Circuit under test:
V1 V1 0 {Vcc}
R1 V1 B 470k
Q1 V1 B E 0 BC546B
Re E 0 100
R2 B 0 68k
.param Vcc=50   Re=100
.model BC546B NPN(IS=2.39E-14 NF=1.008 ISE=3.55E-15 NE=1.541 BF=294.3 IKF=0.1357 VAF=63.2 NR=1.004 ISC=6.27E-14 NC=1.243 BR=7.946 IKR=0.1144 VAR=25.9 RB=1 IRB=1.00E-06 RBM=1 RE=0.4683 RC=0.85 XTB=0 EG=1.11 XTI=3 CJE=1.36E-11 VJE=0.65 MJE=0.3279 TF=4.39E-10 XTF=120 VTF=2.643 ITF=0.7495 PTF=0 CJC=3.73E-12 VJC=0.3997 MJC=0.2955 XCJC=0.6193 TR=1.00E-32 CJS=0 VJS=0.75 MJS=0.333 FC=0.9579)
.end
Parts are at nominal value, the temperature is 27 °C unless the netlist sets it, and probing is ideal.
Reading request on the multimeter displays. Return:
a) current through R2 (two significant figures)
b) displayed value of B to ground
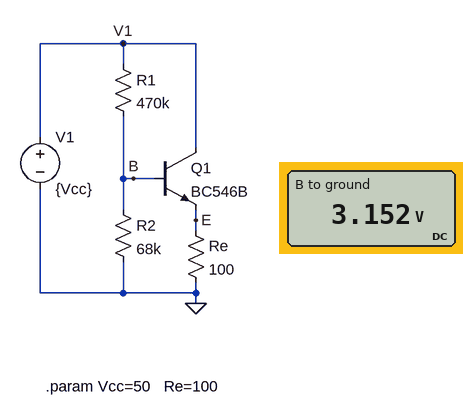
46 µA
3.152 V
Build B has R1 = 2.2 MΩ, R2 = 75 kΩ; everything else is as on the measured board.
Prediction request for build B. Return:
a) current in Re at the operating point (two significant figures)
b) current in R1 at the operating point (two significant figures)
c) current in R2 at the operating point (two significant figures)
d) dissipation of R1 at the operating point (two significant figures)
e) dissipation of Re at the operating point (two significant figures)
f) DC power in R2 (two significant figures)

4.0 mA
22 µA
14 µA
1.1 mW
1.6 mW
15 µW
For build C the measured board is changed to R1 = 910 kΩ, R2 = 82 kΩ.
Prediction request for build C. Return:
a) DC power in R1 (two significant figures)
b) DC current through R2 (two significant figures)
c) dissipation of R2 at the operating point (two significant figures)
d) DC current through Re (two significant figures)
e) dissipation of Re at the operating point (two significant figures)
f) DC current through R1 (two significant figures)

2.5 mW
25 µA
51 µW
13 mA
18 mW
53 µA
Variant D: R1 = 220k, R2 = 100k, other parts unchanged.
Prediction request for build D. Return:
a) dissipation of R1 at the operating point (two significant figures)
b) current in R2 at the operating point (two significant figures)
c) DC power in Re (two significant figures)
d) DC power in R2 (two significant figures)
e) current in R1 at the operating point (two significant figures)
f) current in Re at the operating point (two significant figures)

8.7 mW
62 µA
290 mW
380 µW
200 µA
54 mA
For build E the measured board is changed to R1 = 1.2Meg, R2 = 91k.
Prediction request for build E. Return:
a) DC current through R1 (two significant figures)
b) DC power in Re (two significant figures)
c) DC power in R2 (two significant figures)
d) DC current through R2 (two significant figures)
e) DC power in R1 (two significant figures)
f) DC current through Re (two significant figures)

40 µA
11 mW
33 µW
19 µA
1.9 mW
10 mA
